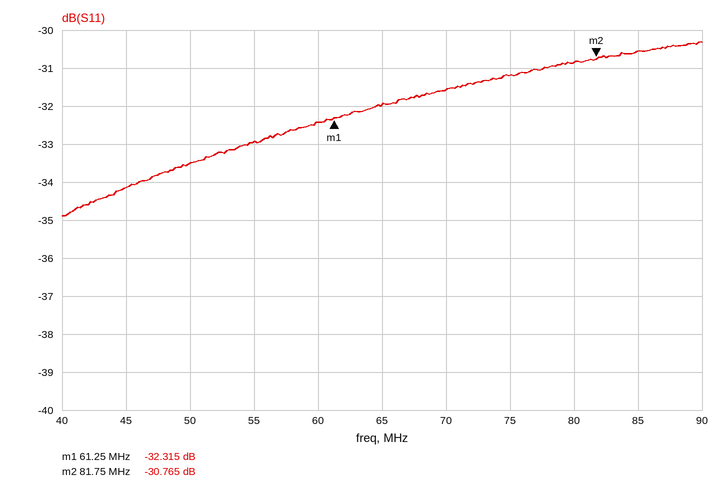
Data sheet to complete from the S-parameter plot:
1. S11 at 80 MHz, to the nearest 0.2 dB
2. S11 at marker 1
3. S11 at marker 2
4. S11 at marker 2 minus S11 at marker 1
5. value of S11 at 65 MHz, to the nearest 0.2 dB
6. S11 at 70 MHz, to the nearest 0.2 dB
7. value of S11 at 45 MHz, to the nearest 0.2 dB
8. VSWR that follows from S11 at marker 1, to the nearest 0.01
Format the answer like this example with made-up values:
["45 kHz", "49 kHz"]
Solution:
["-30.8 dB", "-32.315 dB", "-30.765 dB", "1.550 dB", "-32.0 dB", "-31.6 dB", "-34.2 dB", "1.05"]
